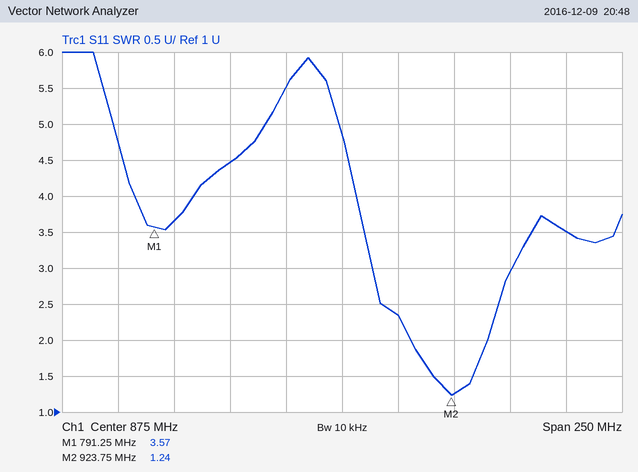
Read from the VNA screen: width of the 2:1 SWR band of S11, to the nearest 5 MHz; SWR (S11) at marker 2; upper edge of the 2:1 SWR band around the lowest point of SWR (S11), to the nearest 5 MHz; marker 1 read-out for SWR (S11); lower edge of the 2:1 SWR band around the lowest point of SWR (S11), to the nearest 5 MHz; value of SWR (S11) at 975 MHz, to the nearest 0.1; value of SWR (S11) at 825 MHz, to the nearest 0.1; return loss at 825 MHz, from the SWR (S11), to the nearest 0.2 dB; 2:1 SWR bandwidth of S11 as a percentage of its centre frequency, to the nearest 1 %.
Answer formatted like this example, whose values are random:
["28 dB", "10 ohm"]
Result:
["35 MHz", "1.24", "940 MHz", "3.57", "905 MHz", "3.5", "4.5", "4.0 dB", "4 %"]
